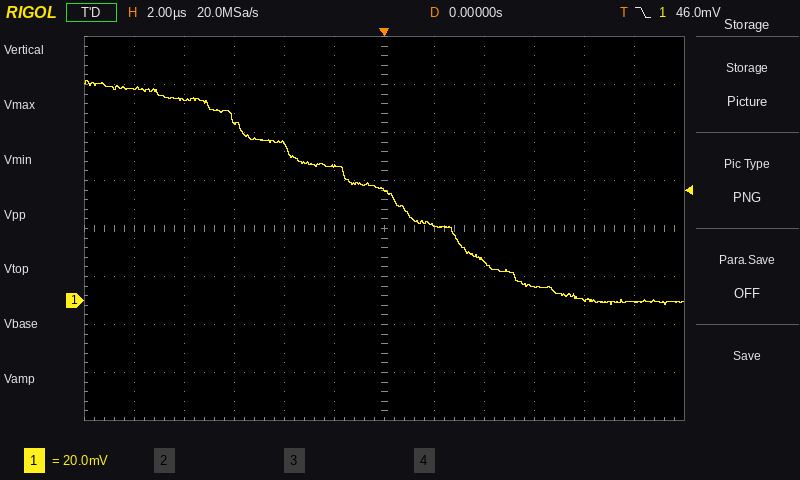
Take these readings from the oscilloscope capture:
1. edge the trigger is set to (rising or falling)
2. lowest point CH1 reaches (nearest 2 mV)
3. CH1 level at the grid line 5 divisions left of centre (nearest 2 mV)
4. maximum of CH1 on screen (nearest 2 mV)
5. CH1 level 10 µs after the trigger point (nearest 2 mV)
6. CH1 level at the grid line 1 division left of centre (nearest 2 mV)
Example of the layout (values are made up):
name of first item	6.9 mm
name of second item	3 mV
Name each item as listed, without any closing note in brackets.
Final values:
edge the trigger is set to	falling
lowest point CH1 reaches	-2 mV
CH1 level at the grid line 5 divisions left of centre	88 mV
maximum of CH1 on screen	92 mV
CH1 level 10 µs after the trigger point	0 mV
CH1 level at the grid line 1 division left of centre	56 mV
